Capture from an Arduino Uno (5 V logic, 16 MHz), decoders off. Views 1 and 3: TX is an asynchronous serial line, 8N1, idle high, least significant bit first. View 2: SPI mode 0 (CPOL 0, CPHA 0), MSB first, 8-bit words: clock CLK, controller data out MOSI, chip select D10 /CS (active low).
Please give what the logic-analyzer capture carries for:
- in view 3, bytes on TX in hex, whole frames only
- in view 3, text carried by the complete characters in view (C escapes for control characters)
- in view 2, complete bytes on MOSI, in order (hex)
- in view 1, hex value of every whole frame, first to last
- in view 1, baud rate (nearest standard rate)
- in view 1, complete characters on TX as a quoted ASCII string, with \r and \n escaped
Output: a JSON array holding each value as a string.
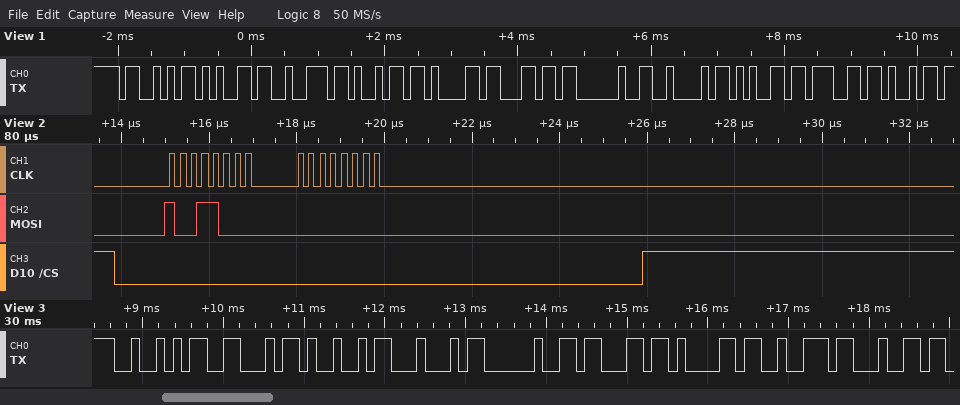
["52 46 49 44 20 63 61 72 64", "\"RFID card\"", "98 00", "53 65 72 69 61 6C 20 42 65 67 69", "9600 baud", "\"Serial Begi\""]
